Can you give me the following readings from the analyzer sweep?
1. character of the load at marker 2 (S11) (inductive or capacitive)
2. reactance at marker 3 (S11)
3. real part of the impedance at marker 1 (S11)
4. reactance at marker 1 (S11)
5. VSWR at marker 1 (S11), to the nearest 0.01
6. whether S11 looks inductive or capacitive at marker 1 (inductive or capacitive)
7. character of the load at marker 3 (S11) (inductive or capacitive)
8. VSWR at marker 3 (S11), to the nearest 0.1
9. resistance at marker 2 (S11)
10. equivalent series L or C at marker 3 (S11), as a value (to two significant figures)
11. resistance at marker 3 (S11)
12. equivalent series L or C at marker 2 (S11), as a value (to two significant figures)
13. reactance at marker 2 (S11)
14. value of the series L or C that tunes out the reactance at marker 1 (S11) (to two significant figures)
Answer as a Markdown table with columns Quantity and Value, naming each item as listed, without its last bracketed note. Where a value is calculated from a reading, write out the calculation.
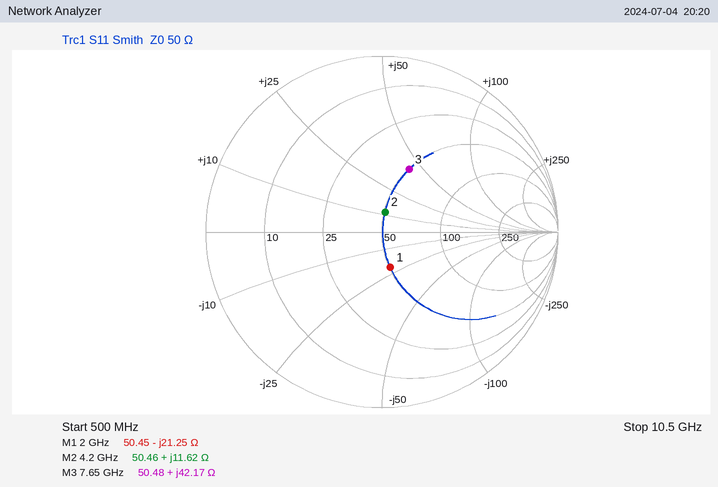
| Quantity | Value |
|---|---|
| character of the load at marker 2 (S11) | inductive |
| reactance at marker 3 | +42.17 Ω |
| real part of the impedance at marker 1 | 50.45 Ω |
| reactance at marker 1 | -21.25 Ω |
| VSWR at marker 1 (S11), to the nearest 0.01 | 1.52 |
| whether S11 looks inductive or capacitive at marker 1 | capacitive |
| character of the load at marker 3 (S11) | inductive |
| VSWR at marker 3 (S11), to the nearest 0.1 | 2.3 |
| resistance at marker 2 | 50.46 Ω |
| equivalent series L or C at marker 3 (S11), as a value | L = 42.17 Ω/(2π × 7.65 GHz) ≈ 877 pH, so 880 pH to two significant figures |
| resistance at marker 3 | 50.48 Ω |
| equivalent series L or C at marker 2 (S11), as a value | L = 11.62 Ω/(2π × 4.2 GHz) ≈ 440 pH |
| reactance at marker 2 | +11.62 Ω |
| value of the series L or C that tunes out the reactance at marker 1 (S11) | L = 21.25 Ω/(2π × 2 GHz) ≈ 1.7 nH |
